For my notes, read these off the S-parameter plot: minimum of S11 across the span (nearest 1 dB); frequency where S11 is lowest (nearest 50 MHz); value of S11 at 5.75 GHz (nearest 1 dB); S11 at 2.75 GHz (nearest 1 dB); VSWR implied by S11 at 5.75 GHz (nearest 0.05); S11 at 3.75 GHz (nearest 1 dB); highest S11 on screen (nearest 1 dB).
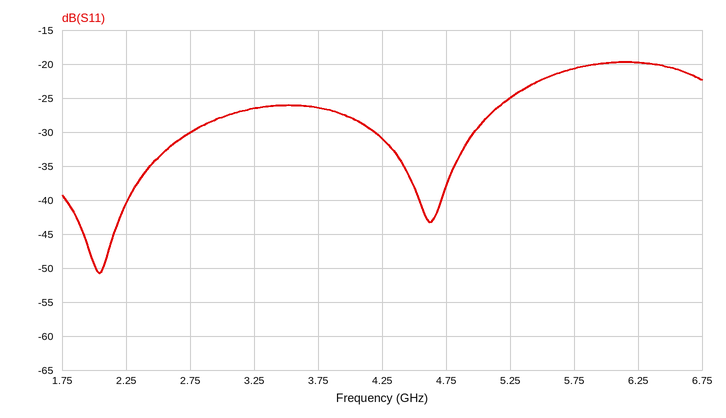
-51 dB
2.05 GHz
-21 dB
-30 dB
1.20
-26 dB
-20 dB
